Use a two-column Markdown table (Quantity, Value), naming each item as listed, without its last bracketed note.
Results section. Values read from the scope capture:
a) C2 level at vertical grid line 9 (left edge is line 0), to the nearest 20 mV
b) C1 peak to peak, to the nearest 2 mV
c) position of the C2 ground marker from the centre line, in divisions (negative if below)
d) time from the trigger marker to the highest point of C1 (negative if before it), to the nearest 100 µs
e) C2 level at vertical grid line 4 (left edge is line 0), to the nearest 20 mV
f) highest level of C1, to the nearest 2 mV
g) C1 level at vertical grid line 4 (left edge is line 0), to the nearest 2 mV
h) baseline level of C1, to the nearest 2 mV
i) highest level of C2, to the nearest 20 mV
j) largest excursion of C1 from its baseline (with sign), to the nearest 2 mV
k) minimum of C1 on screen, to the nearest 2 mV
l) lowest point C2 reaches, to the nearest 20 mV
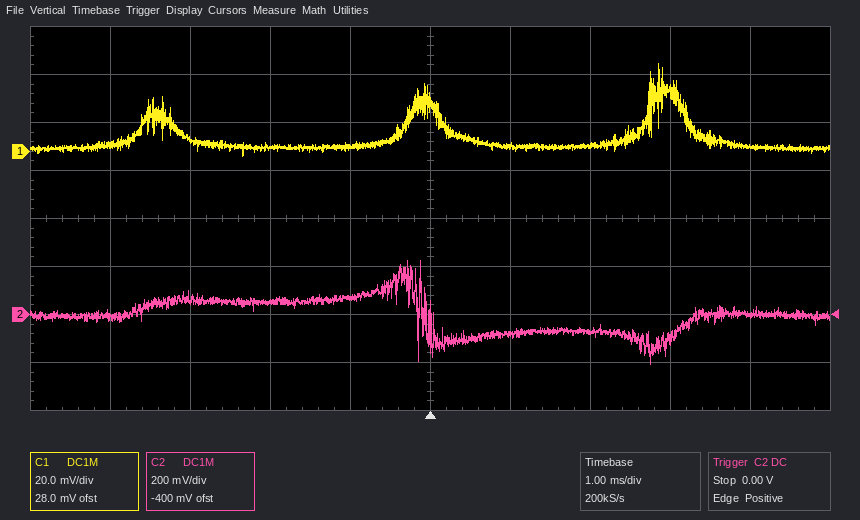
| Quantity | Value |
|---|---|
| C2 level at vertical grid line 9 (left edge is line 0), to the nearest 20 mV | 0 mV |
| C1 peak to peak, to the nearest 2 mV | 38 mV |
| position of the C2 ground marker from the centre line, in divisions | -2.0 div |
| time from the trigger marker to the highest point of C1 (negative if before it), to the nearest 100 µs | +2.9 ms |
| C2 level at vertical grid line 4 (left edge is line 0), to the nearest 20 mV | 80 mV |
| highest level of C1, to the nearest 2 mV | 36 mV |
| C1 level at vertical grid line 4 (left edge is line 0), to the nearest 2 mV | 2 mV |
| baseline level of C1, to the nearest 2 mV | 2 mV |
| highest level of C2, to the nearest 20 mV | 220 mV |
| largest excursion of C1 from its baseline (with sign), to the nearest 2 mV | +34 mV |
| minimum of C1 on screen, to the nearest 2 mV | -2 mV |
| lowest point C2 reaches, to the nearest 20 mV | -200 mV |
